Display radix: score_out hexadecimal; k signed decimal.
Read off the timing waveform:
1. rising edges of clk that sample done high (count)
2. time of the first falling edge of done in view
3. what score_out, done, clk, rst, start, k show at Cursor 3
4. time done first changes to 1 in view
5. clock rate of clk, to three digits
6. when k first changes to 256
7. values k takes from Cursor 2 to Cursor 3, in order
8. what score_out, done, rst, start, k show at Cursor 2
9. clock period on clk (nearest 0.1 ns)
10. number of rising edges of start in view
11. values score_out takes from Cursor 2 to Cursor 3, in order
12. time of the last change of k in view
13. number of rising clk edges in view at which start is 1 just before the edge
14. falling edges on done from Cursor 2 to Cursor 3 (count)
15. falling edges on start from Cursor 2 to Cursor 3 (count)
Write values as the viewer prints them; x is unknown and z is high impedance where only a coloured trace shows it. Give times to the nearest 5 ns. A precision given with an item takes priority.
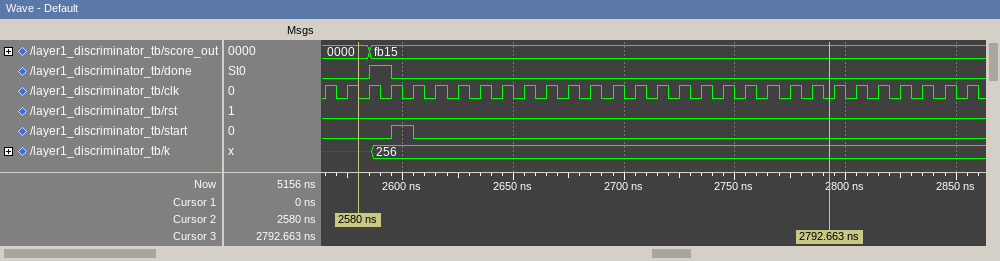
1
2595 ns
score_out=fb15, done=0, clk=0, rst=0, start=0, k=256
2585 ns
100 MHz
2585 ns
x, 256
score_out=0000, done=0, rst=0, start=0, k=x
10 ns
1
0000, fb15
2585 ns
1
1
1
